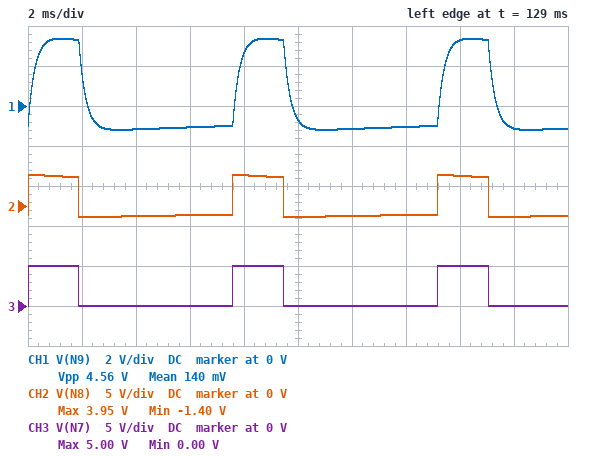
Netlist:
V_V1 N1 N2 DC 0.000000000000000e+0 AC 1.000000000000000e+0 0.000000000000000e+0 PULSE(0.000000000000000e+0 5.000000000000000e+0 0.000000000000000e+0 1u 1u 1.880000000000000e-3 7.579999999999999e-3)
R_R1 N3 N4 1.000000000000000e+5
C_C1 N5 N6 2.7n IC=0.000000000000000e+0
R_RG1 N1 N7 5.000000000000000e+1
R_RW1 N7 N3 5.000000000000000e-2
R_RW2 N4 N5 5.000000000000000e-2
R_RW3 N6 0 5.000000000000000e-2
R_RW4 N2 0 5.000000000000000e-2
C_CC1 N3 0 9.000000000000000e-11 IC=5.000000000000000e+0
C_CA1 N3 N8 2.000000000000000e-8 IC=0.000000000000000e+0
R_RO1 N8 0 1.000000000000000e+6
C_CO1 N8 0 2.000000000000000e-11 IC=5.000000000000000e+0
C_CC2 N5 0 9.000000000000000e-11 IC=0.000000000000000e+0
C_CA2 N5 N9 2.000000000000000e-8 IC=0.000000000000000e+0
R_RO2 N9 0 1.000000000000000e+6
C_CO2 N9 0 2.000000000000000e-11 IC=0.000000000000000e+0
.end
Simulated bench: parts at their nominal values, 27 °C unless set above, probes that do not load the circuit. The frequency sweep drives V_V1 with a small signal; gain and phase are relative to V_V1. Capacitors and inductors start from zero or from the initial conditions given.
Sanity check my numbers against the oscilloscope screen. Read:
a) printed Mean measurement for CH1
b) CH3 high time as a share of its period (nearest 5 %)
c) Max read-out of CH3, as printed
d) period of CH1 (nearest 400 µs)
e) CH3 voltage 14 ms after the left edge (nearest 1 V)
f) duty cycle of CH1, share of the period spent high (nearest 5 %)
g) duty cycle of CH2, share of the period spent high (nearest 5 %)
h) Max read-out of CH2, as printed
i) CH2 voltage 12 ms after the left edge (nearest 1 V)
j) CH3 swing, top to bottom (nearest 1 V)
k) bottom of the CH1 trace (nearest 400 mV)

140 mV
25 %
5.00 V
7.6 ms
0 V
25 %
25 %
3.95 V
-1 V
5 V
-1.2 V
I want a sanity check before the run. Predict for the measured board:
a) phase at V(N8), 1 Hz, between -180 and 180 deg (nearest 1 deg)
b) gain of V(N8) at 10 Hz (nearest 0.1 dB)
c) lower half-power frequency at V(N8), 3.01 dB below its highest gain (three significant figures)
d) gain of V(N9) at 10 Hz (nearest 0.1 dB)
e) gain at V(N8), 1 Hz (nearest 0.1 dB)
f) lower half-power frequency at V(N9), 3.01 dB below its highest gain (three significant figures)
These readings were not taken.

83 deg
-2.1 dB
7.94 Hz
-2.7 dB
-18.1 dB
7.06 Hz
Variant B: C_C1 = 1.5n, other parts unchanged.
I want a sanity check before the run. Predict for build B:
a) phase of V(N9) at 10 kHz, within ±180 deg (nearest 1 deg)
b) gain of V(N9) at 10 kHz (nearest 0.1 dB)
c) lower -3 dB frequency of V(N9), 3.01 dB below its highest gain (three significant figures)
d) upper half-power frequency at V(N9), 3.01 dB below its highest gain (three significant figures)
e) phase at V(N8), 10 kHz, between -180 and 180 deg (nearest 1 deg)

-84 deg
-20.2 dB
7.13 Hz
1.10 kHz
0 deg
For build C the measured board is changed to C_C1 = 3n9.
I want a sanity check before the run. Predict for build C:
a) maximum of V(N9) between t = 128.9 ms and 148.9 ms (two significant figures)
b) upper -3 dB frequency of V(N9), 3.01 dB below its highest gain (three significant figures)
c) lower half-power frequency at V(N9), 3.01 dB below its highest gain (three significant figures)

3.3 V
451 Hz
6.99 Hz
